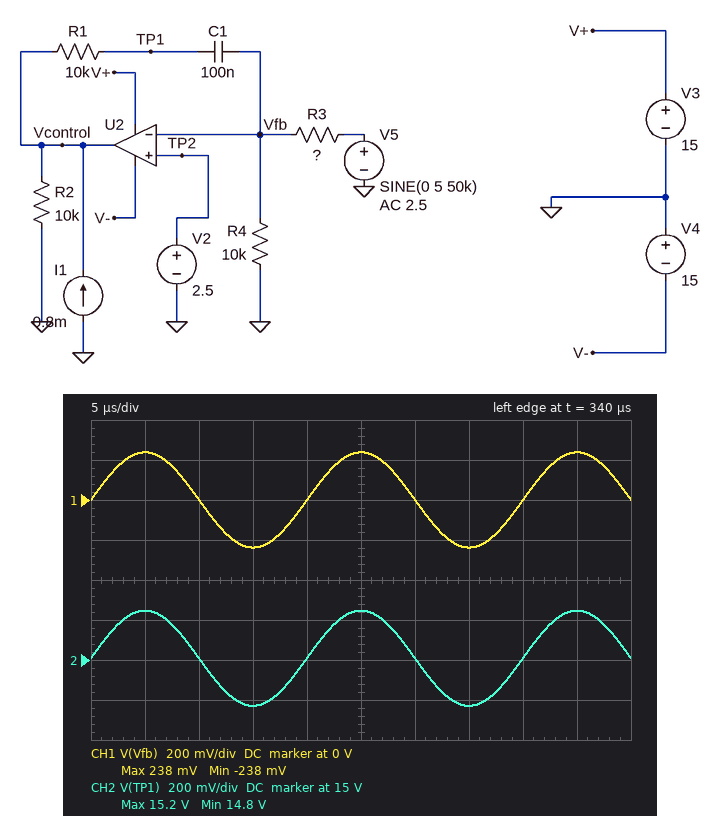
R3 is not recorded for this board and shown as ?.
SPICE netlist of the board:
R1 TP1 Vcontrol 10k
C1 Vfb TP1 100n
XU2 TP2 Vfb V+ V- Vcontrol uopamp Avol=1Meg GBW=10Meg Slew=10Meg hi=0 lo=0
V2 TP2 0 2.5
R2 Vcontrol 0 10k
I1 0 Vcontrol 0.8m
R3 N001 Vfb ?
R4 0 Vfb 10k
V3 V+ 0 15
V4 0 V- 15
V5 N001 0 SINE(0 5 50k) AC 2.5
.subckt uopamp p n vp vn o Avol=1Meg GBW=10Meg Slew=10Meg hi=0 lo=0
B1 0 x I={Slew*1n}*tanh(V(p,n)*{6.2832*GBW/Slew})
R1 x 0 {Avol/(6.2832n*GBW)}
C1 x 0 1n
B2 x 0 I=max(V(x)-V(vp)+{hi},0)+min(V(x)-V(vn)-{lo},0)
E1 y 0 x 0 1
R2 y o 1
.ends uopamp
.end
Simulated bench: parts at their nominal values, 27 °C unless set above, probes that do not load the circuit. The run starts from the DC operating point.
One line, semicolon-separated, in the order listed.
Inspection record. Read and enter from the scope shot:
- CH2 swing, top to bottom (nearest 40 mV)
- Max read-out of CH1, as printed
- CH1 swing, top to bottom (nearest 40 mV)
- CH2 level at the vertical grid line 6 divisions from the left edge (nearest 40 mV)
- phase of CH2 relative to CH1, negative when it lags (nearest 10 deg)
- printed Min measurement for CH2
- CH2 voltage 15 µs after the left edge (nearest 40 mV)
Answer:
480 mV; 238 mV; 480 mV; 15.00 V; 0 deg; 14.8 V; 14.76 V
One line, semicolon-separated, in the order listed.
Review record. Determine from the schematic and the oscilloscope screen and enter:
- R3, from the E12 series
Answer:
100 kΩ
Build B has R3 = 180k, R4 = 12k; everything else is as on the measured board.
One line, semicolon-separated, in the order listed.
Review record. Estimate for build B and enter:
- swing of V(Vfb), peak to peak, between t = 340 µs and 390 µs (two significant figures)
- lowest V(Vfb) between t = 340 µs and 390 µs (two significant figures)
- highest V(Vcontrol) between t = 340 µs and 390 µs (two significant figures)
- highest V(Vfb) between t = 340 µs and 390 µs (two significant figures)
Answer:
290 mV; -150 mV; 15 V; 150 mV
